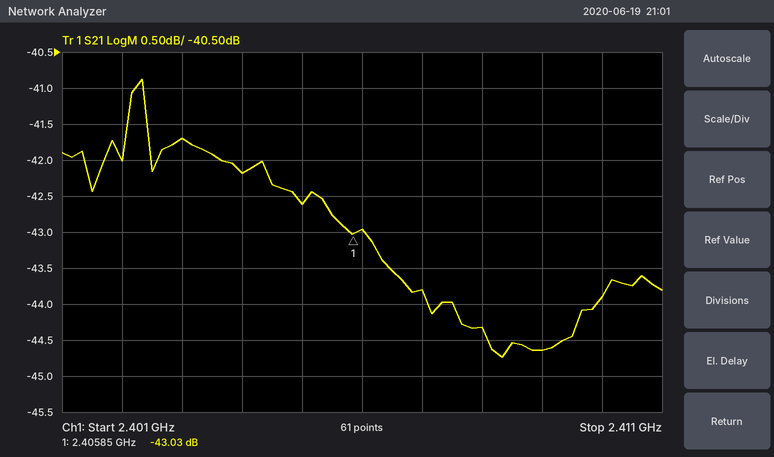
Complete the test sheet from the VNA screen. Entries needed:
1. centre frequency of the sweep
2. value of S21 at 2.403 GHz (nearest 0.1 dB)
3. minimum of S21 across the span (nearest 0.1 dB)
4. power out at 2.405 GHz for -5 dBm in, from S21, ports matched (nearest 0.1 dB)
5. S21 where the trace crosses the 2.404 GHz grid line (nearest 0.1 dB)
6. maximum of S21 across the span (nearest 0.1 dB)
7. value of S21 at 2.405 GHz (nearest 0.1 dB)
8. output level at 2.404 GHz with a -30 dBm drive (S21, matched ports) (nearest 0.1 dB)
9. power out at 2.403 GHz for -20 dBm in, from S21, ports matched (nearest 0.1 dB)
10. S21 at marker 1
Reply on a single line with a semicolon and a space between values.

2.406 GHz; -41.7 dB; -44.7 dB; -47.6 dBm; -42.2 dB; -40.9 dB; -42.6 dB; -72.2 dBm; -61.7 dBm; -43.03 dB
